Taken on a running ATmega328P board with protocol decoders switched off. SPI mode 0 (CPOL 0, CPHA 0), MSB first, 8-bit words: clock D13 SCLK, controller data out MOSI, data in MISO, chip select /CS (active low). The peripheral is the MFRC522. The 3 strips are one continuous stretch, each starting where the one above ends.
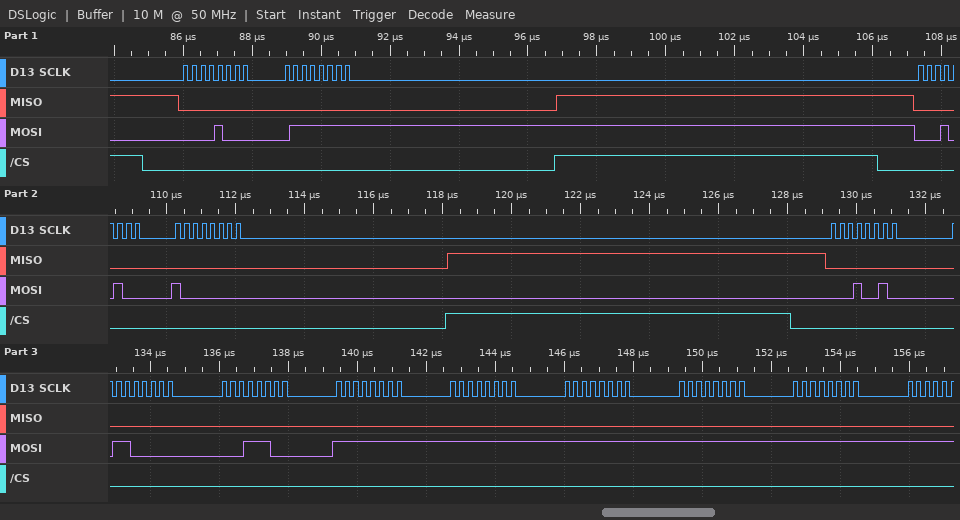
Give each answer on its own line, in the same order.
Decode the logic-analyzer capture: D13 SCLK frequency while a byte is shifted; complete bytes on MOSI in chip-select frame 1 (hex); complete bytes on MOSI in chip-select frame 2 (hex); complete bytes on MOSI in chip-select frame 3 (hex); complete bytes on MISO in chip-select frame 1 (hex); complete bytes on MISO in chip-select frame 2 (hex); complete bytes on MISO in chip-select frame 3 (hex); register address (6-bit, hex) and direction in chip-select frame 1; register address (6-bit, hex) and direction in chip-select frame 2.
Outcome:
4 MHz
08 7F
14 80
12 60 1C FF FF FF FF FF
00 00
00 00
00 00 00 00 00 00 00 00
0x04 write
0x0A write
